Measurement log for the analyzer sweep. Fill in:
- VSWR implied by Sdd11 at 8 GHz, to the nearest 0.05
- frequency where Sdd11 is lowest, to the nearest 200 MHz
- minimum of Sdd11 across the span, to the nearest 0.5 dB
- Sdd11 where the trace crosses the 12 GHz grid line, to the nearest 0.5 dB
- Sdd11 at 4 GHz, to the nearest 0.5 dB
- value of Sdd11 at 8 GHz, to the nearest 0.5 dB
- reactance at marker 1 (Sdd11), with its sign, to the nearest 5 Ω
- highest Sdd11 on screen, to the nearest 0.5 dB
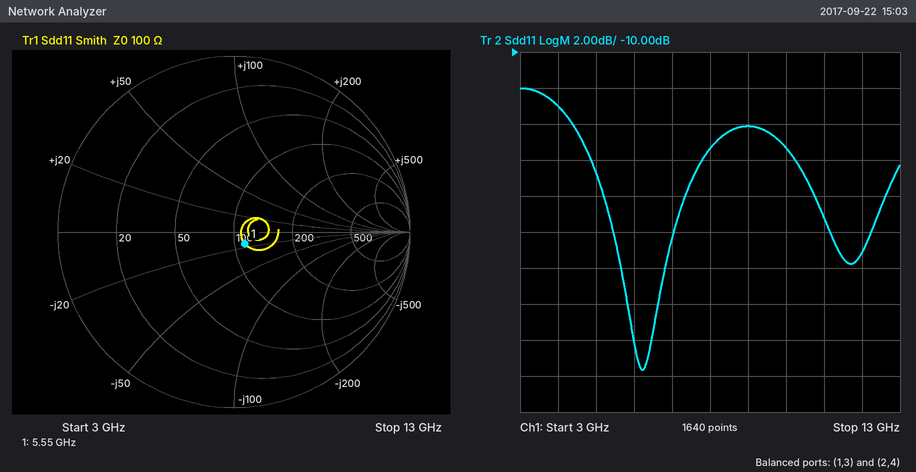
1.40
6.2 GHz
-27.5 dB
-21.0 dB
-13.0 dB
-15.5 dB
-15 Ω
-12.0 dB
